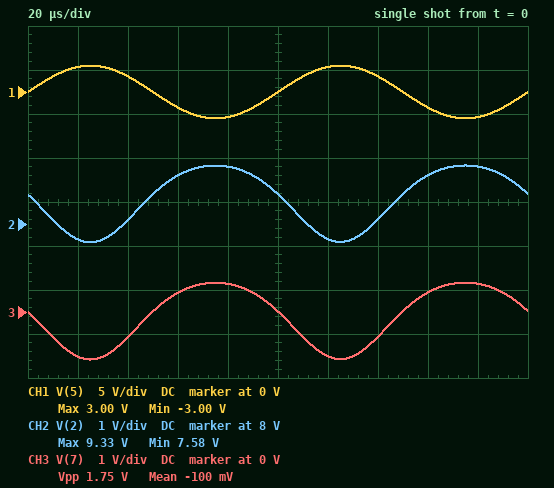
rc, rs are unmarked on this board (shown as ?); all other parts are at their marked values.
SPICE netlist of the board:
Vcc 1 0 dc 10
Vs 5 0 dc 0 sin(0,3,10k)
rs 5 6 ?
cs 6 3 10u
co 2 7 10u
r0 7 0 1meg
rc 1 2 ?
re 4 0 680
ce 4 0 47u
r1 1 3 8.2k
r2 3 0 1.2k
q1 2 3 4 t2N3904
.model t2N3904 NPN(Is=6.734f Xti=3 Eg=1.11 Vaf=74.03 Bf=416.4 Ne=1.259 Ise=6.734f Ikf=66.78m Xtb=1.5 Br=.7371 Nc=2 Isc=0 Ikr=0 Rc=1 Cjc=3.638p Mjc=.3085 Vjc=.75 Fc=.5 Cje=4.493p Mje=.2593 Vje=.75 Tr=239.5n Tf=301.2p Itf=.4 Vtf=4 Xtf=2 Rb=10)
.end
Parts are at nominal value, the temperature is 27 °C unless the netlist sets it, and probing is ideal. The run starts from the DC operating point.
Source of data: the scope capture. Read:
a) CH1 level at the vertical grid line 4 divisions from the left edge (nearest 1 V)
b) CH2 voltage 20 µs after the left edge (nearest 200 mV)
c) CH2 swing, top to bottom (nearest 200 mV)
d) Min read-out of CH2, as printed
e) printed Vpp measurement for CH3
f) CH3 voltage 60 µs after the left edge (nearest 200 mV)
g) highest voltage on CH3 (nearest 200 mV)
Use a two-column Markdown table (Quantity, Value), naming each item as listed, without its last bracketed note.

| Quantity | Value |
|---|---|
| CH1 level at the vertical grid line 4 divisions from the left edge | -3 V |
| CH2 voltage 20 µs after the left edge | 7.6 V |
| CH2 swing, top to bottom | 1.8 V |
| Min read-out of CH2, as printed | 7.58 V |
| printed Vpp measurement for CH3 | 1.75 V |
| CH3 voltage 60 µs after the left edge | 400 mV |
| highest voltage on CH3 | 600 mV |
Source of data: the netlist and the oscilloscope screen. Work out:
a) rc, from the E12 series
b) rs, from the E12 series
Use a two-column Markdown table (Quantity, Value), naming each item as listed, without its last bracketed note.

| Quantity | Value |
|---|---|
| rc, from the E12 series | 1.5 kΩ |
| rs, from the E12 series | 150 kΩ |
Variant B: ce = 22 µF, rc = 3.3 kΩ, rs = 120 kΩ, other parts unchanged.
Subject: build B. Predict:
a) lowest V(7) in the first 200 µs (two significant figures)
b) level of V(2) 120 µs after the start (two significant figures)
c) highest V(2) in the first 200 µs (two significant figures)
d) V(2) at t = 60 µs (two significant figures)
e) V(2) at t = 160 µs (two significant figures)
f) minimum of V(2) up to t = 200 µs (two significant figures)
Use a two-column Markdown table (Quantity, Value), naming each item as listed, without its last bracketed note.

| Quantity | Value |
|---|---|
| lowest V(7) in the first 200 µs | -2.9 V |
| level of V(2) 120 µs after the start | 4.4 V |
| highest V(2) in the first 200 µs | 8.8 V |
| V(2) at t = 60 µs | 8.2 V |
| V(2) at t = 160 µs | 8.3 V |
| minimum of V(2) up to t = 200 µs | 4.1 V |
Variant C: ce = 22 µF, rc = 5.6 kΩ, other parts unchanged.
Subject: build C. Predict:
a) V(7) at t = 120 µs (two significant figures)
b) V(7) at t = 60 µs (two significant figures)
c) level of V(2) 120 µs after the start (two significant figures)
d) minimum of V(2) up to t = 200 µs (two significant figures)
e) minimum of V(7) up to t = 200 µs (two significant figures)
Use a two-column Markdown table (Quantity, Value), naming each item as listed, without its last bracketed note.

| Quantity | Value |
|---|---|
| V(7) at t = 120 µs | -3.3 V |
| V(7) at t = 60 µs | 1.6 V |
| level of V(2) 120 µs after the start | 1.7 V |
| minimum of V(2) up to t = 200 µs | 1.4 V |
| minimum of V(7) up to t = 200 µs | -3.6 V |
